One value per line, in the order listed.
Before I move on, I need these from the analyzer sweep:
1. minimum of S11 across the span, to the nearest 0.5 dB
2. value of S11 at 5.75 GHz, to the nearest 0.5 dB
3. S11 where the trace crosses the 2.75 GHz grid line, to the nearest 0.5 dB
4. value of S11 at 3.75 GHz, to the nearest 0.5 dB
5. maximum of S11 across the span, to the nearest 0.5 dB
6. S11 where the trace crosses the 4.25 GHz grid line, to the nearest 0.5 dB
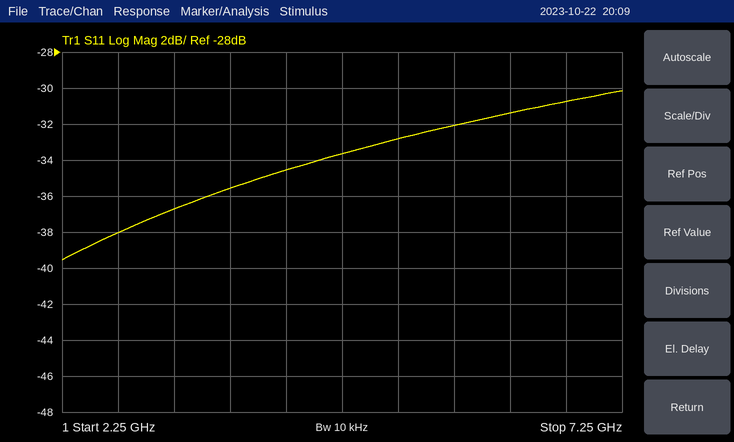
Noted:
-39.5 dB
-32.0 dB
-38.0 dB
-35.5 dB
-30.0 dB
-34.5 dB
